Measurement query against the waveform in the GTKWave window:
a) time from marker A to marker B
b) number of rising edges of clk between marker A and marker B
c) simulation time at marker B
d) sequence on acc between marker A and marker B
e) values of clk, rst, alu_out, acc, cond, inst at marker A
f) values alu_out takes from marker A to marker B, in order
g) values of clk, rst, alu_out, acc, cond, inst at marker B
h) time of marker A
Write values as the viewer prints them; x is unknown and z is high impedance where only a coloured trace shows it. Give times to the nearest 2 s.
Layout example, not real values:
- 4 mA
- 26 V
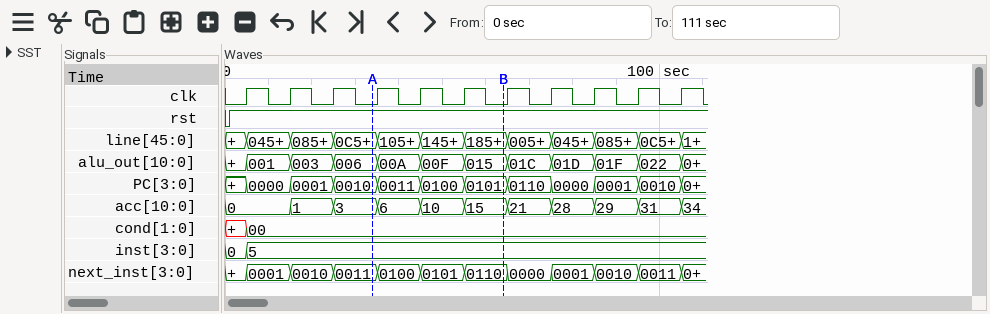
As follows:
- 30 s
- 3
- 64 s
- 3, 6, 10, 15
- clk=0, rst=1, alu_out=006, acc=3, cond=00, inst=5
- 006, 00A, 00F, 015
- clk=0, rst=1, alu_out=015, acc=15, cond=00, inst=5
- 34 s
